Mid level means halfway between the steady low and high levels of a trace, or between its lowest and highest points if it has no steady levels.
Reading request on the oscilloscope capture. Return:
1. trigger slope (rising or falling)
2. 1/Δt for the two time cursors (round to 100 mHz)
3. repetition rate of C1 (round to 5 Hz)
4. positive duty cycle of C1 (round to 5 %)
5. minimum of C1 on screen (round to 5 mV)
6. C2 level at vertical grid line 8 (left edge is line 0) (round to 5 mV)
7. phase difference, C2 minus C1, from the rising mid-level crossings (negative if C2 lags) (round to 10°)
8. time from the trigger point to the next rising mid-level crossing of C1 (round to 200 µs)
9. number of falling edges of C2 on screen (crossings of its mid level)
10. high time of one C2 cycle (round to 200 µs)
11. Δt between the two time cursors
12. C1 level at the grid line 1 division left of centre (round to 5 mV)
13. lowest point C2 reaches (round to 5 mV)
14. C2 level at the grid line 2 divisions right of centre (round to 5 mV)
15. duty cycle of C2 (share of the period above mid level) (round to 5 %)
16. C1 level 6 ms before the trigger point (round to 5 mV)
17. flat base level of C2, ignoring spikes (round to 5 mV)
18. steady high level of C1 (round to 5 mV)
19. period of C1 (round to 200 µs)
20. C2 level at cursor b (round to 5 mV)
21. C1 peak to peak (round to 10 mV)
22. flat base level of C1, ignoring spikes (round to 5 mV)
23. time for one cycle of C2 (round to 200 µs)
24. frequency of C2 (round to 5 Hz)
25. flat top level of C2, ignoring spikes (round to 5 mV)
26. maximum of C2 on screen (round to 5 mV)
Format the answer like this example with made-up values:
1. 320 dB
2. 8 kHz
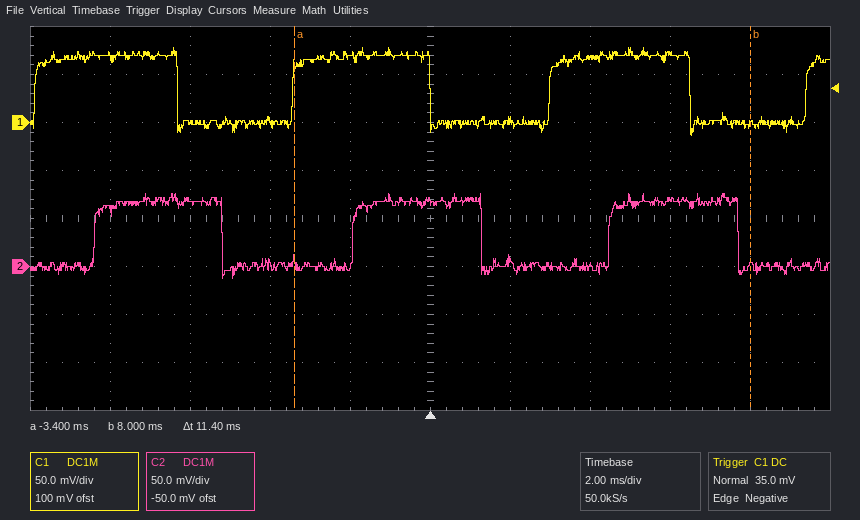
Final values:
1. falling
2. 87.7 Hz
3. 155 Hz
4. 55 %
5. -15 mV
6. 70 mV
7. -80°
8. 3.0 ms
9. 3
10. 3.2 ms
11. 11.4 ms
12. 70 mV
13. -10 mV
14. 0 mV
15. 50 %
16. 0 mV
17. 0 mV
18. 70 mV
19. 6.4 ms
20. 0 mV
21. 90 mV
22. 0 mV
23. 6.4 ms
24. 155 Hz
25. 70 mV
26. 75 mV
